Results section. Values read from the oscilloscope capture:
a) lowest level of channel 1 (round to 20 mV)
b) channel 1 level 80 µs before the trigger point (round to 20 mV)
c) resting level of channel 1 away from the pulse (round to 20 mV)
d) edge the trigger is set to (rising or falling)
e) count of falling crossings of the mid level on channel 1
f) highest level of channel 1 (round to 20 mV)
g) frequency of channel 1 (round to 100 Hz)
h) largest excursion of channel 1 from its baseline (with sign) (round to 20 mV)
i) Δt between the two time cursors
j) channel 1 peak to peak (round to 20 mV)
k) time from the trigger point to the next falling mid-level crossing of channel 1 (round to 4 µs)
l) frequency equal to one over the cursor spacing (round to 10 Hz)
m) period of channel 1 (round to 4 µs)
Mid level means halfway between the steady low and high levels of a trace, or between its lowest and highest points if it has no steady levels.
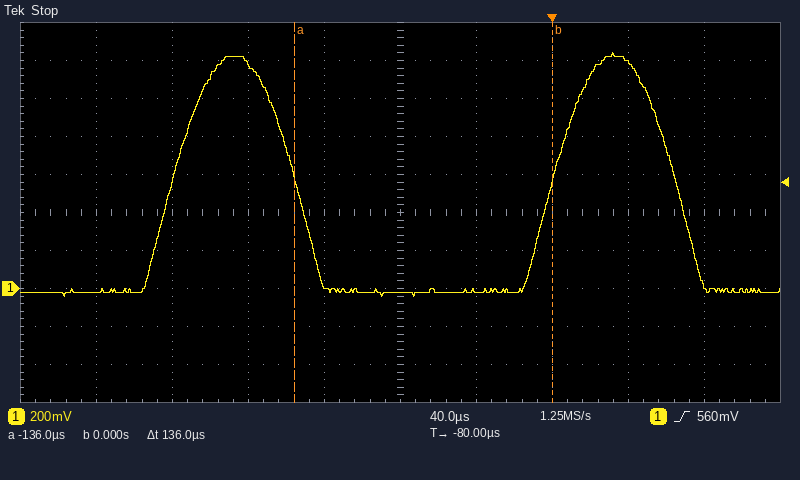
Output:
-40 mV
-20 mV
-20 mV
rising
2
1.24 V
5.0 kHz
+1.26 V
136 µs
1.28 V
64 µs
7.35 kHz
200 µs
